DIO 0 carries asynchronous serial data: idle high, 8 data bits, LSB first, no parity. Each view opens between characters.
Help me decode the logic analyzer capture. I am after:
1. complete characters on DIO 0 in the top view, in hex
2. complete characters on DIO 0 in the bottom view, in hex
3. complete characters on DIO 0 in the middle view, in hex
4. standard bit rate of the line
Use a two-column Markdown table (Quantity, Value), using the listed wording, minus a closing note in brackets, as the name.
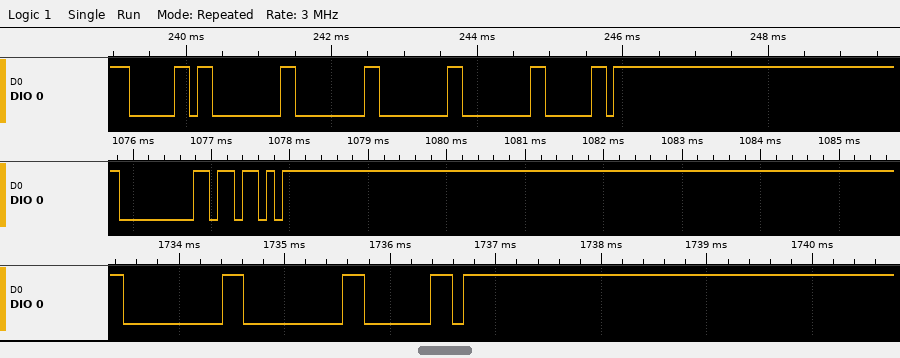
| Quantity | Value |
|---|---|
| complete characters on DIO 0 in the top view, in hex | 60, 00, 00, 00, 00, 60 |
| complete characters on DIO 0 in the bottom view, in hex | 00, 00, 60 |
| complete characters on DIO 0 in the middle view, in hex | 00, 5B |
| standard bit rate of the line | 9600 baud |
